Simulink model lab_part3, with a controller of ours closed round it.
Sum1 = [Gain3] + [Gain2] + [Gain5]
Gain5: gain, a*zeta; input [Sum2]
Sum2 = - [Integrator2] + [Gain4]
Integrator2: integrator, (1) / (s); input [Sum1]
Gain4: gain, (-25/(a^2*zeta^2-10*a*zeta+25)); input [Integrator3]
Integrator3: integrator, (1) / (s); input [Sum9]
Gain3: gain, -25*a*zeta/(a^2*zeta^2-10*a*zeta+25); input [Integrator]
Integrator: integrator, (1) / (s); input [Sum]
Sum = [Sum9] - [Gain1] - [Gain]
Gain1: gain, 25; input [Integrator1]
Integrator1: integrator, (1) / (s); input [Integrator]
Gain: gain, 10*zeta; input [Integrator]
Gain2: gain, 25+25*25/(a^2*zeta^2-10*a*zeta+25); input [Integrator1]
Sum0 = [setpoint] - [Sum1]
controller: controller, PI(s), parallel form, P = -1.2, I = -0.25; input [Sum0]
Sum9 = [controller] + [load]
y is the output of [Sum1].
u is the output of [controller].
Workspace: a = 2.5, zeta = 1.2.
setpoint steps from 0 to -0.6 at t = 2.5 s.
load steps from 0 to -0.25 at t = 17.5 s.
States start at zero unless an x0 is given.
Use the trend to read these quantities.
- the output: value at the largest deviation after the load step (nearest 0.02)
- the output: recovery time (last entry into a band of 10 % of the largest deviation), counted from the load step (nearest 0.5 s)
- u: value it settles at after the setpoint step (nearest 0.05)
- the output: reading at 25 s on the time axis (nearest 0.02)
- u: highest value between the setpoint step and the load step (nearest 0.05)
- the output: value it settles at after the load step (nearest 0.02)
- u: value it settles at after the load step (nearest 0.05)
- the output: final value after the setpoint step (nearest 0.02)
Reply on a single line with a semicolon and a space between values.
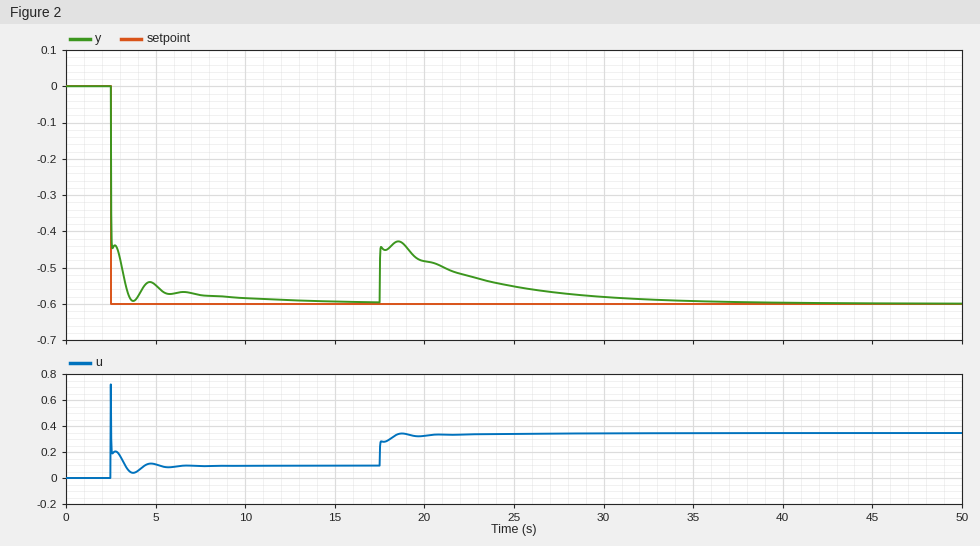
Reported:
-0.42; 13.0 s; 0.10; -0.56; 0.70; -0.60; 0.35; -0.60
